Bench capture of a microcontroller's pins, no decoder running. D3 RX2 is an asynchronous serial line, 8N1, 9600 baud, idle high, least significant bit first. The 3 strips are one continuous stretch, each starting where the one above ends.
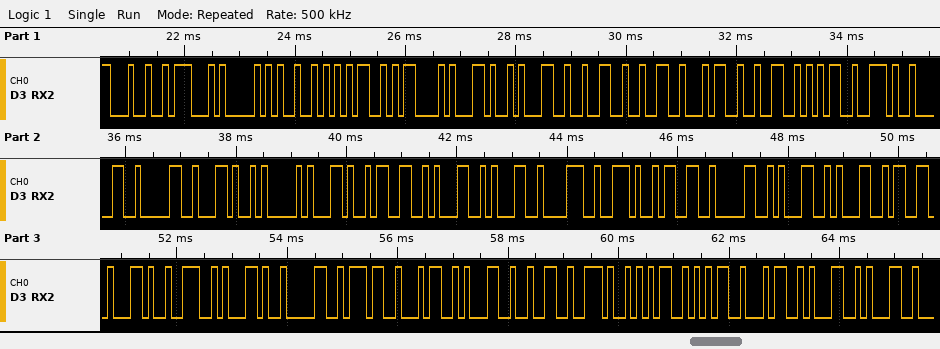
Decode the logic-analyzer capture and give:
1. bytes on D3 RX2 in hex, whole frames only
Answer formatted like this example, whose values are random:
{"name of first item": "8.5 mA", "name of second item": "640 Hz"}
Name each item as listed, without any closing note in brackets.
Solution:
{"bytes on D3 RX2 in hex, whole frames only": "24 47 50 52 4D 43 2C 31 32 32 34 32 35 2E 30 30 2C 41 2C 33 31 31 38 2E 33 30 31 31 33 2C 4E 2C 30 37 34 31 32 2E 35 35 34 31 31"}
